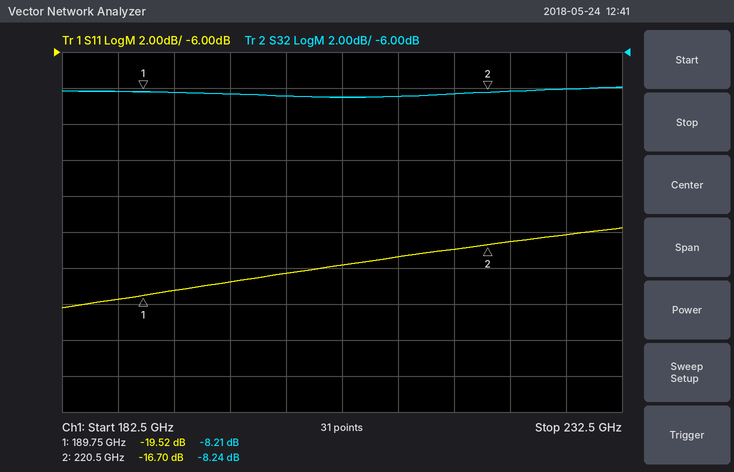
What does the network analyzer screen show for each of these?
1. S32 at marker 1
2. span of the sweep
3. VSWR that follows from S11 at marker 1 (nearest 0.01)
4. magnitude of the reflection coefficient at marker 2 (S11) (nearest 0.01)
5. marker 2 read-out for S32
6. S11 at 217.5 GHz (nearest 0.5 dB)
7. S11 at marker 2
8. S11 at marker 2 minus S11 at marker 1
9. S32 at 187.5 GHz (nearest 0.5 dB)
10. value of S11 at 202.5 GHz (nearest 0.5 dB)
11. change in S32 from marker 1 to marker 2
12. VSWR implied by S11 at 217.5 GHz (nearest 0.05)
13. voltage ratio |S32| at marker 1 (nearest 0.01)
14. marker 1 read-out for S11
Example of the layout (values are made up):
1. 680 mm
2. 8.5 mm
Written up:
1. -8.21 dB
2. 50 GHz
3. 1.24
4. 0.15
5. -8.24 dB
6. -17.0 dB
7. -16.70 dB
8. 2.82 dB
9. -8.0 dB
10. -18.5 dB
11. -0.03 dB
12. 1.35
13. 0.39
14. -19.52 dB
